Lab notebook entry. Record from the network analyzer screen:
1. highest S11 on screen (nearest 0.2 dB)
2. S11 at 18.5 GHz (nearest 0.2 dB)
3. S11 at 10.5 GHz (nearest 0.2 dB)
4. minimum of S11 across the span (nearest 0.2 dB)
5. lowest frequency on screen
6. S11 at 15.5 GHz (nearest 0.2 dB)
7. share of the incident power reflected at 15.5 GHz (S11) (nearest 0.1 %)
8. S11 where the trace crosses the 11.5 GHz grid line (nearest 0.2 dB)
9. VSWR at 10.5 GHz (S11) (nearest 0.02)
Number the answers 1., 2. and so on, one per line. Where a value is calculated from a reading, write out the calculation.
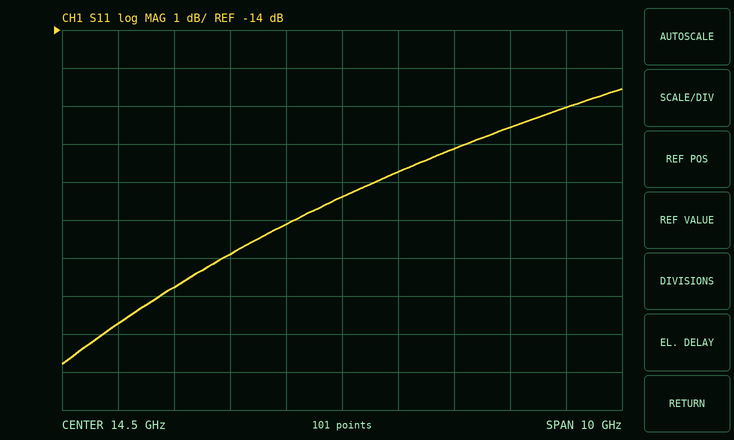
1. -15.6 dB
2. -16.0 dB
3. -21.8 dB
4. -22.8 dB
5. 9.5 GHz
6. -17.8 dB
7. 10^(-17.8/10) ≈ 1.7 %
8. -20.8 dB
9. |Γ| = 10^(-21.8/20) = 0.0813; VSWR = (1 + 0.0813)/(1 − 0.0813) ≈ 1.18
